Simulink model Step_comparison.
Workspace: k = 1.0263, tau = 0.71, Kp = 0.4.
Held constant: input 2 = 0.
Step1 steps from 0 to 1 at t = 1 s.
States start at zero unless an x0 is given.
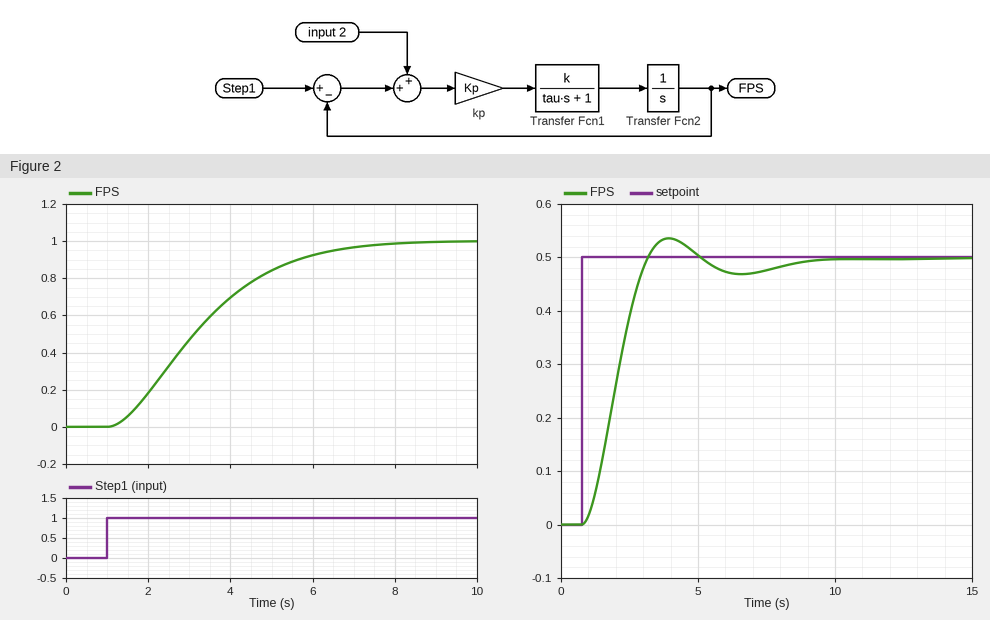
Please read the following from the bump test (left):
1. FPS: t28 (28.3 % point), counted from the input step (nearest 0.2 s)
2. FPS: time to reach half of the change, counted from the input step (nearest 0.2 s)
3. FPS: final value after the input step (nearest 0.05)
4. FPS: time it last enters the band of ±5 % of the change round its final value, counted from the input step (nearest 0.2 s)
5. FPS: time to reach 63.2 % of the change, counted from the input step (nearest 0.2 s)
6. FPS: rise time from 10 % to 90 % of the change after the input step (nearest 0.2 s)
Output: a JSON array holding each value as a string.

["1.4 s", "2.2 s", "1.00", "5.6 s", "2.6 s", "4.0 s"]
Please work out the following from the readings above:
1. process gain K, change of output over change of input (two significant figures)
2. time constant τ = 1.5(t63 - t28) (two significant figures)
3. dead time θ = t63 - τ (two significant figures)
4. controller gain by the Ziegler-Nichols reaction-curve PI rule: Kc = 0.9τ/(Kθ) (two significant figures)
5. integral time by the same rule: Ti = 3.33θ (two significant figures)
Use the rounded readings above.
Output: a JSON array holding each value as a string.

["1.0", "1.8 s", "0.80 s", "2.0", "2.7 s"]
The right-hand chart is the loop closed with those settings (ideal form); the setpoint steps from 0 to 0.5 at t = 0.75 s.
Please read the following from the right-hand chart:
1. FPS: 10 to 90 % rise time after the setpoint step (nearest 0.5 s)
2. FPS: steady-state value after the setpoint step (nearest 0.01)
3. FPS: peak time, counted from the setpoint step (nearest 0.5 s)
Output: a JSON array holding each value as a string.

["1.5 s", "0.50", "3.0 s"]
